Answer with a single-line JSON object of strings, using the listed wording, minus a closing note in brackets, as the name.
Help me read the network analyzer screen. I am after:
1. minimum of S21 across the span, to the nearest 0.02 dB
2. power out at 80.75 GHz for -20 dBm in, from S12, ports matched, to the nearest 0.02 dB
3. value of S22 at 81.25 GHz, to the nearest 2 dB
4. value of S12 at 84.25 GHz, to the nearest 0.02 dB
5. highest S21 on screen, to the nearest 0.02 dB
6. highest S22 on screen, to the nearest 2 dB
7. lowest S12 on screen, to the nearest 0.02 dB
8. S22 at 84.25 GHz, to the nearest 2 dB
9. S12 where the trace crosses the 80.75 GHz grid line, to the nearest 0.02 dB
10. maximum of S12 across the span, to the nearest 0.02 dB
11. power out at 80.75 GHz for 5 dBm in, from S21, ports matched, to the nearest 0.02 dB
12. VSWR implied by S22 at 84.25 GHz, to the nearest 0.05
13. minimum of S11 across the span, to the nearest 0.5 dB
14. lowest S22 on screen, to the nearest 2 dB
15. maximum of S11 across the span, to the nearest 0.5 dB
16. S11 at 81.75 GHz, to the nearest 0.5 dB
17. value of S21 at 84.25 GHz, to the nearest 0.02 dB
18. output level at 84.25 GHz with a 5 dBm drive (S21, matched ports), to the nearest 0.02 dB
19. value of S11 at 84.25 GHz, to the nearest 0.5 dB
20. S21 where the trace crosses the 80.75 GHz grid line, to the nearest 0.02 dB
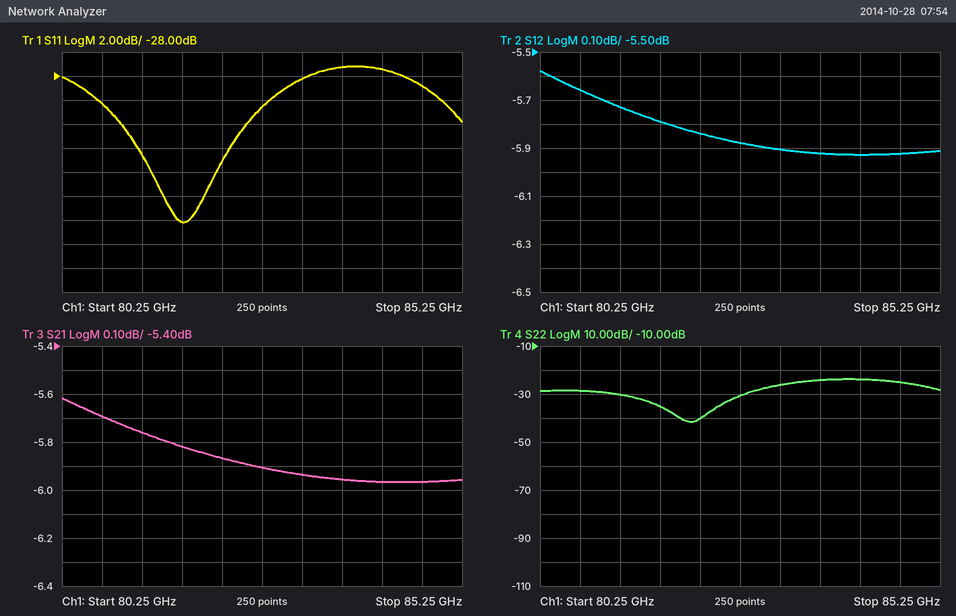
{"minimum of S21 across the span, to the nearest 0.02 dB": "-5.96 dB", "power out at 80.75 GHz for -20 dBm in, from S12, ports matched, to the nearest 0.02 dB": "-25.66 dBm", "value of S22 at 81.25 GHz, to the nearest 2 dB": "-30 dB", "value of S12 at 84.25 GHz, to the nearest 0.02 dB": "-5.92 dB", "highest S21 on screen, to the nearest 0.02 dB": "-5.62 dB", "highest S22 on screen, to the nearest 2 dB": "-24 dB", "lowest S12 on screen, to the nearest 0.02 dB": "-5.92 dB", "S22 at 84.25 GHz, to the nearest 2 dB": "-24 dB", "S12 where the trace crosses the 80.75 GHz grid line, to the nearest 0.02 dB": "-5.66 dB", "maximum of S12 across the span, to the nearest 0.02 dB": "-5.58 dB", "power out at 80.75 GHz for 5 dBm in, from S21, ports matched, to the nearest 0.02 dB": "-0.70 dBm", "VSWR implied by S22 at 84.25 GHz, to the nearest 0.05": "1.15", "minimum of S11 across the span, to the nearest 0.5 dB": "-40.0 dB", "lowest S22 on screen, to the nearest 2 dB": "-42 dB", "maximum of S11 across the span, to the nearest 0.5 dB": "-27.0 dB", "S11 at 81.75 GHz, to the nearest 0.5 dB": "-40.0 dB", "value of S21 at 84.25 GHz, to the nearest 0.02 dB": "-5.96 dB", "output level at 84.25 GHz with a 5 dBm drive (S21, matched ports), to the nearest 0.02 dB": "-0.96 dBm", "value of S11 at 84.25 GHz, to the nearest 0.5 dB": "-27.5 dB", "S21 where the trace crosses the 80.75 GHz grid line, to the nearest 0.02 dB": "-5.70 dB"}
